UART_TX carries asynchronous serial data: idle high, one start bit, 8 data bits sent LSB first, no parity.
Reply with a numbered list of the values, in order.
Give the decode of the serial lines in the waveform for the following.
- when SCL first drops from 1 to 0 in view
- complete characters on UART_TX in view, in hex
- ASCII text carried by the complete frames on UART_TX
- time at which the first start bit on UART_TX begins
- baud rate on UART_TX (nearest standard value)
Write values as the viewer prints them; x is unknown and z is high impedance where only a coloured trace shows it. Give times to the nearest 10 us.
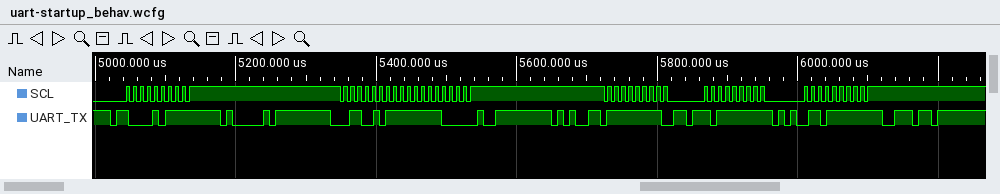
1. 5050 us
2. 43, 41, 4C, 20, 65, 76, 65, 6E
3. "CAL even"
4. 5020 us
5. 115200 baud
